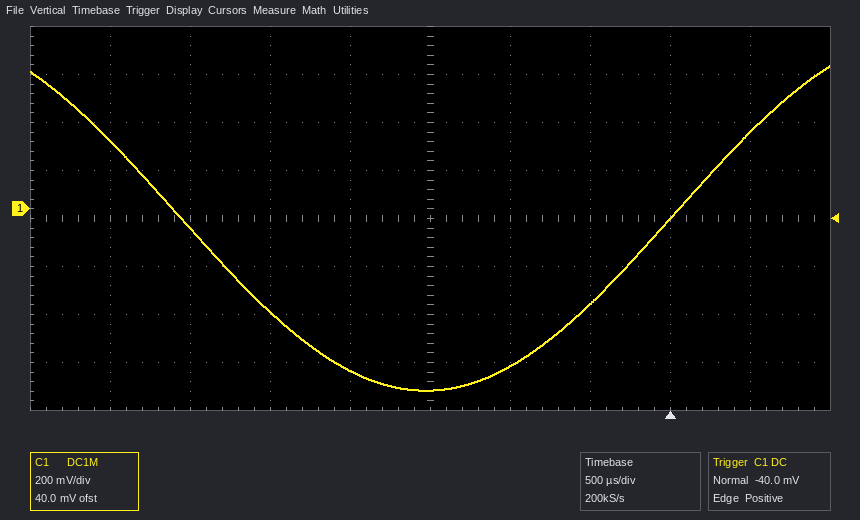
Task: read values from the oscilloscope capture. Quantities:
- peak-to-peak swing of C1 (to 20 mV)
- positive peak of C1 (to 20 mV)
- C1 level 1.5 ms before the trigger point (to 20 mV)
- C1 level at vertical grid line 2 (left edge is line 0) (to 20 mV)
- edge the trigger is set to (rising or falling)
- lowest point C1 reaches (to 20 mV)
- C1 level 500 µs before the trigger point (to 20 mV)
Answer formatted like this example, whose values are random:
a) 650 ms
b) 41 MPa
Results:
a) 1.36 V
b) 600 mV
c) -760 mV
d) -80 mV
e) rising
f) -760 mV
g) -400 mV
